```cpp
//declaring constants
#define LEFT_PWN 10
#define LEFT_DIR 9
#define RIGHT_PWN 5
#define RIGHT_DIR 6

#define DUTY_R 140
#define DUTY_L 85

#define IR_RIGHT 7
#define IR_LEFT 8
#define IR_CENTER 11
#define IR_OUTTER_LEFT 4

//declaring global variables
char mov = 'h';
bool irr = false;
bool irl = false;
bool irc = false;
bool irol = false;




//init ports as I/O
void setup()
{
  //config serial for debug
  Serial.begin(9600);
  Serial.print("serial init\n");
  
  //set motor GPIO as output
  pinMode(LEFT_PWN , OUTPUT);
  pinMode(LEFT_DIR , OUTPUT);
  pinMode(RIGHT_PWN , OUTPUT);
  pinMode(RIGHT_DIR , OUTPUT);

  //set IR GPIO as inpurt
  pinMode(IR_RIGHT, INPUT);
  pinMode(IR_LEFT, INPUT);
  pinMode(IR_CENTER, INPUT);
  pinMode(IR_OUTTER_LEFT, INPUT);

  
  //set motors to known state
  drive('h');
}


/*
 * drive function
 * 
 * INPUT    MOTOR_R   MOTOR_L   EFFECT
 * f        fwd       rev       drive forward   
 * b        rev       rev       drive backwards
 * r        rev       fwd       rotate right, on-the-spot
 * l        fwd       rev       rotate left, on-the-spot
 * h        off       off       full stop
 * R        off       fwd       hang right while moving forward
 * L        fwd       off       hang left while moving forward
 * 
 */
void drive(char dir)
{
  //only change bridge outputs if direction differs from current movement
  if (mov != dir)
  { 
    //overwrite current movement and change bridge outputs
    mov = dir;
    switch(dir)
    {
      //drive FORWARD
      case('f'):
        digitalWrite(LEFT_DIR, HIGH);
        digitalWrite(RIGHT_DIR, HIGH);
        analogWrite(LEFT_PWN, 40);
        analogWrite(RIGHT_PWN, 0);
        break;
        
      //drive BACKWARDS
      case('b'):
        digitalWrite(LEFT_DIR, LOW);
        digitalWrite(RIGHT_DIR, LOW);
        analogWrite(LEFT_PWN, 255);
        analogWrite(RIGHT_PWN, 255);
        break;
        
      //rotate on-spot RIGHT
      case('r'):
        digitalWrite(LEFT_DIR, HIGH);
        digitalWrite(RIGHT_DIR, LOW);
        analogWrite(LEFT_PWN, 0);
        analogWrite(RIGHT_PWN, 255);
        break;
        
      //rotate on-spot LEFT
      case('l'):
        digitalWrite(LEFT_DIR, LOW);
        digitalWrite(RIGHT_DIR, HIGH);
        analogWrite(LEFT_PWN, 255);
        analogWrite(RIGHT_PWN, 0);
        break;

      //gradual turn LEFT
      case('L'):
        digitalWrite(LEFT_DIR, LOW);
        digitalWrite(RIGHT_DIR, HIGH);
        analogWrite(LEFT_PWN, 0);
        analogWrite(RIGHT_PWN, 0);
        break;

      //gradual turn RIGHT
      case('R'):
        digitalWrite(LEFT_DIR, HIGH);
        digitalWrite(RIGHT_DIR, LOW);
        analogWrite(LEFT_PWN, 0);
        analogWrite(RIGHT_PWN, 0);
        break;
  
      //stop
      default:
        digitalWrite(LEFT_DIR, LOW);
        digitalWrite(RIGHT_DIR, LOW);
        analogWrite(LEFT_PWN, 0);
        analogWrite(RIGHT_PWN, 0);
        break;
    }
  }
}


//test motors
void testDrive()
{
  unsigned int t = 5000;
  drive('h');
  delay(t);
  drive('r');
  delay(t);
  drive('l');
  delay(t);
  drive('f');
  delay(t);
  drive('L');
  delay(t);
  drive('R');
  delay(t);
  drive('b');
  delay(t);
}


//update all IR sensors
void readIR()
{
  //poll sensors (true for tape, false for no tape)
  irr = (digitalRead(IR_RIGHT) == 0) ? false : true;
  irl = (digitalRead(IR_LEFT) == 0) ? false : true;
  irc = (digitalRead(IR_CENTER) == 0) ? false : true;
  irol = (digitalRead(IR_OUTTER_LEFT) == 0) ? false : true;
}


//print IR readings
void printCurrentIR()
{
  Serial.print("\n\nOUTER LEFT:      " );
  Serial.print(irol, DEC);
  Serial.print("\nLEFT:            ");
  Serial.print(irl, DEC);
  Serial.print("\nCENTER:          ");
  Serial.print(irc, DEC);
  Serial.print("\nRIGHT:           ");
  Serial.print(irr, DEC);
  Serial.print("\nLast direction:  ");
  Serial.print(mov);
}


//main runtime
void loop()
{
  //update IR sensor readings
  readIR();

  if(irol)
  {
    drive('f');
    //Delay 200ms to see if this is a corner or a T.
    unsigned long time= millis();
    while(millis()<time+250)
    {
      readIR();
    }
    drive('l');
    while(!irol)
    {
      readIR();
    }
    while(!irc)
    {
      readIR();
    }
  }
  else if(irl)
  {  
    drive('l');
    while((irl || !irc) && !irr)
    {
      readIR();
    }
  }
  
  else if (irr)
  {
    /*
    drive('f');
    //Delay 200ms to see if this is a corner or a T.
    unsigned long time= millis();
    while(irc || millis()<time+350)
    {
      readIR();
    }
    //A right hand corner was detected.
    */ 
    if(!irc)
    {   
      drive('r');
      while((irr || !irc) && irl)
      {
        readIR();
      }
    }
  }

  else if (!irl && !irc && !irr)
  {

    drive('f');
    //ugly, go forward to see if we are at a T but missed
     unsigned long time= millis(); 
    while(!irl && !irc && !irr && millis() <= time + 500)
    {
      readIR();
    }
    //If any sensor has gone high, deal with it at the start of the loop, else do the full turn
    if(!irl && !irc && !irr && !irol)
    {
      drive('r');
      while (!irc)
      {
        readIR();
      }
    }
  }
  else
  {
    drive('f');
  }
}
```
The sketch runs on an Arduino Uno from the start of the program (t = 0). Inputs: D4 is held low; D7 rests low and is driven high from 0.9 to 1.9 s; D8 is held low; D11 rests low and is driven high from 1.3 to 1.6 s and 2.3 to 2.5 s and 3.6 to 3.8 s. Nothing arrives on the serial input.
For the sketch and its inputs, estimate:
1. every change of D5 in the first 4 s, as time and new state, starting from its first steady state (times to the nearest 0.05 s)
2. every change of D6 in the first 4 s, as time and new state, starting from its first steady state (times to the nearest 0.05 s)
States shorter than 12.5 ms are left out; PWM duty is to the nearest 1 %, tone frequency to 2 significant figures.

0 s low; 0.5 s high; 1.9 s low; 3 s high; 3.6 s low
0 s high; 0.5 s low; 1.9 s high; 3 s low; 3.6 s high
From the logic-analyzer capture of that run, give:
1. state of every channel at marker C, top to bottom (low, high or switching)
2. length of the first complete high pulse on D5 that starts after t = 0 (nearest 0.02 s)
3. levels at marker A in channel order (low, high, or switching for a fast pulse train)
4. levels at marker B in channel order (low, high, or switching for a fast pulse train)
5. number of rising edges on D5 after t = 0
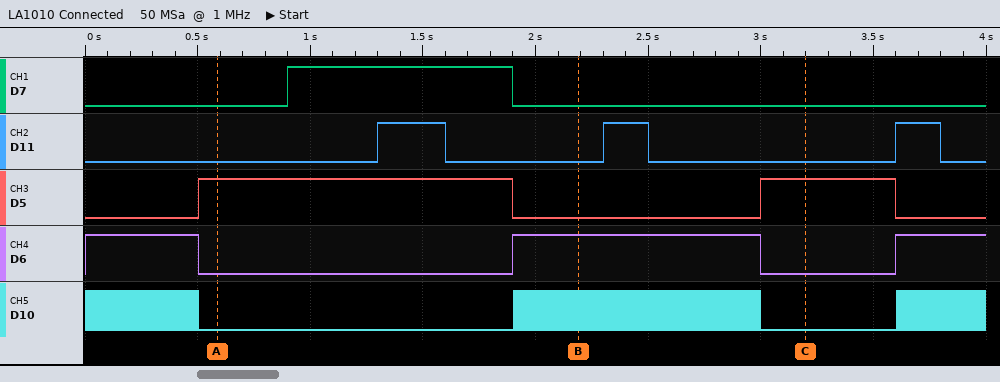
D7 low, D11 low, D5 high, D6 low, D10 low
1.40 s
D7 low, D11 low, D5 high, D6 low, D10 low
D7 low, D11 low, D5 low, D6 high, D10 switching
2
